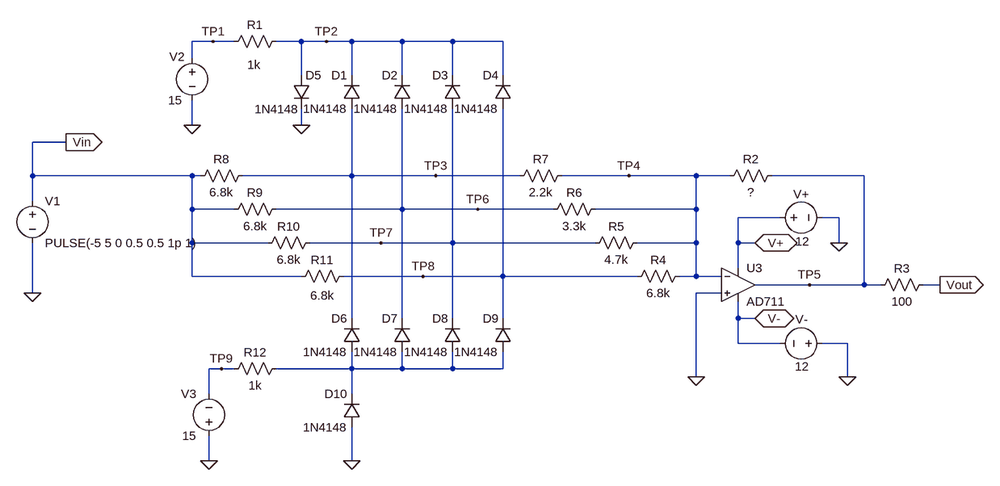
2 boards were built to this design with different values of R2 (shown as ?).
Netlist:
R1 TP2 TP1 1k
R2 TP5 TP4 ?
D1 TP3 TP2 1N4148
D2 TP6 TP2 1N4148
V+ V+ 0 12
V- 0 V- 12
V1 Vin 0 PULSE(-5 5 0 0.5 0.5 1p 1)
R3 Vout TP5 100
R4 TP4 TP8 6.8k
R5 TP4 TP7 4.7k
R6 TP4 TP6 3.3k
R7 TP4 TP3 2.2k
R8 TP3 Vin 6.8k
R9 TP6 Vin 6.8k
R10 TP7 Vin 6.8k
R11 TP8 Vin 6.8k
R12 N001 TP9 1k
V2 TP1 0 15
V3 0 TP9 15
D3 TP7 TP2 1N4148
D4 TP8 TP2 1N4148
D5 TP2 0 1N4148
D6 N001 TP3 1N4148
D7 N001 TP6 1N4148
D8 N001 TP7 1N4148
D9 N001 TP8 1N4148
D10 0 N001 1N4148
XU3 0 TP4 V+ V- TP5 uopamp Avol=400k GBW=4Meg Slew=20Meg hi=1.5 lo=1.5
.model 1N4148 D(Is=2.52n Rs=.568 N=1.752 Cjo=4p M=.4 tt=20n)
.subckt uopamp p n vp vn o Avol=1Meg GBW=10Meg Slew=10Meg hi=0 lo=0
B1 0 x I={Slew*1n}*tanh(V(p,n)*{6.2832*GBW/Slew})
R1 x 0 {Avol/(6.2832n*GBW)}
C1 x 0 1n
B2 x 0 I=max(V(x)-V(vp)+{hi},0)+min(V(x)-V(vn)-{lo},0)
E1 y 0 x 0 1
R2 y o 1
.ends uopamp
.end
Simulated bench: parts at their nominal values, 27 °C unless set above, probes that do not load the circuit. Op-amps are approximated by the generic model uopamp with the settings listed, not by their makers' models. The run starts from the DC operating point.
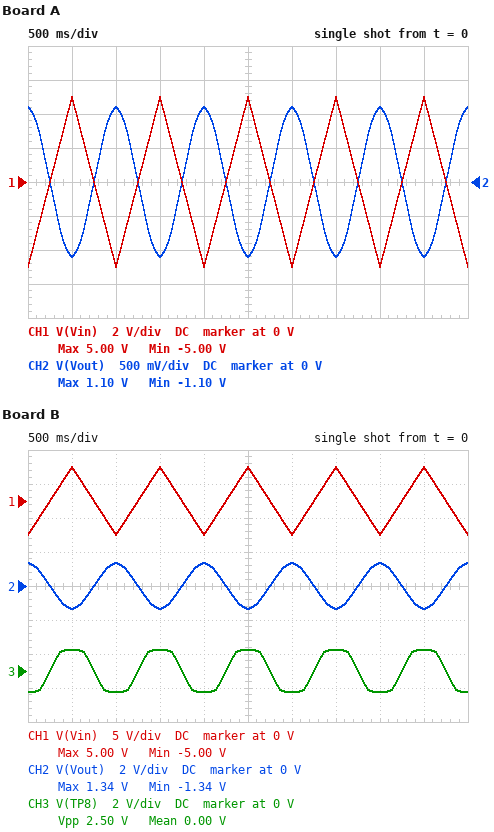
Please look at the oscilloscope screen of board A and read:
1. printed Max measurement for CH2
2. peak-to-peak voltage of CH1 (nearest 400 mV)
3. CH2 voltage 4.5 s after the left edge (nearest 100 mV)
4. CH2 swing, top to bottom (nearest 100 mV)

1.10 V
10.0 V
-1.1 V
2.2 V
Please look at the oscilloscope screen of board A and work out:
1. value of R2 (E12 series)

820 Ω
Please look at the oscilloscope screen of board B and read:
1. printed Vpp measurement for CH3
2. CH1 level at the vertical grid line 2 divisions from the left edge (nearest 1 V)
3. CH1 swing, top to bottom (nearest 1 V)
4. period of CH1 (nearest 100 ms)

2.50 V
-5 V
10 V
1.0 s
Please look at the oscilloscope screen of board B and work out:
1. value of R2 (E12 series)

1 kΩ
